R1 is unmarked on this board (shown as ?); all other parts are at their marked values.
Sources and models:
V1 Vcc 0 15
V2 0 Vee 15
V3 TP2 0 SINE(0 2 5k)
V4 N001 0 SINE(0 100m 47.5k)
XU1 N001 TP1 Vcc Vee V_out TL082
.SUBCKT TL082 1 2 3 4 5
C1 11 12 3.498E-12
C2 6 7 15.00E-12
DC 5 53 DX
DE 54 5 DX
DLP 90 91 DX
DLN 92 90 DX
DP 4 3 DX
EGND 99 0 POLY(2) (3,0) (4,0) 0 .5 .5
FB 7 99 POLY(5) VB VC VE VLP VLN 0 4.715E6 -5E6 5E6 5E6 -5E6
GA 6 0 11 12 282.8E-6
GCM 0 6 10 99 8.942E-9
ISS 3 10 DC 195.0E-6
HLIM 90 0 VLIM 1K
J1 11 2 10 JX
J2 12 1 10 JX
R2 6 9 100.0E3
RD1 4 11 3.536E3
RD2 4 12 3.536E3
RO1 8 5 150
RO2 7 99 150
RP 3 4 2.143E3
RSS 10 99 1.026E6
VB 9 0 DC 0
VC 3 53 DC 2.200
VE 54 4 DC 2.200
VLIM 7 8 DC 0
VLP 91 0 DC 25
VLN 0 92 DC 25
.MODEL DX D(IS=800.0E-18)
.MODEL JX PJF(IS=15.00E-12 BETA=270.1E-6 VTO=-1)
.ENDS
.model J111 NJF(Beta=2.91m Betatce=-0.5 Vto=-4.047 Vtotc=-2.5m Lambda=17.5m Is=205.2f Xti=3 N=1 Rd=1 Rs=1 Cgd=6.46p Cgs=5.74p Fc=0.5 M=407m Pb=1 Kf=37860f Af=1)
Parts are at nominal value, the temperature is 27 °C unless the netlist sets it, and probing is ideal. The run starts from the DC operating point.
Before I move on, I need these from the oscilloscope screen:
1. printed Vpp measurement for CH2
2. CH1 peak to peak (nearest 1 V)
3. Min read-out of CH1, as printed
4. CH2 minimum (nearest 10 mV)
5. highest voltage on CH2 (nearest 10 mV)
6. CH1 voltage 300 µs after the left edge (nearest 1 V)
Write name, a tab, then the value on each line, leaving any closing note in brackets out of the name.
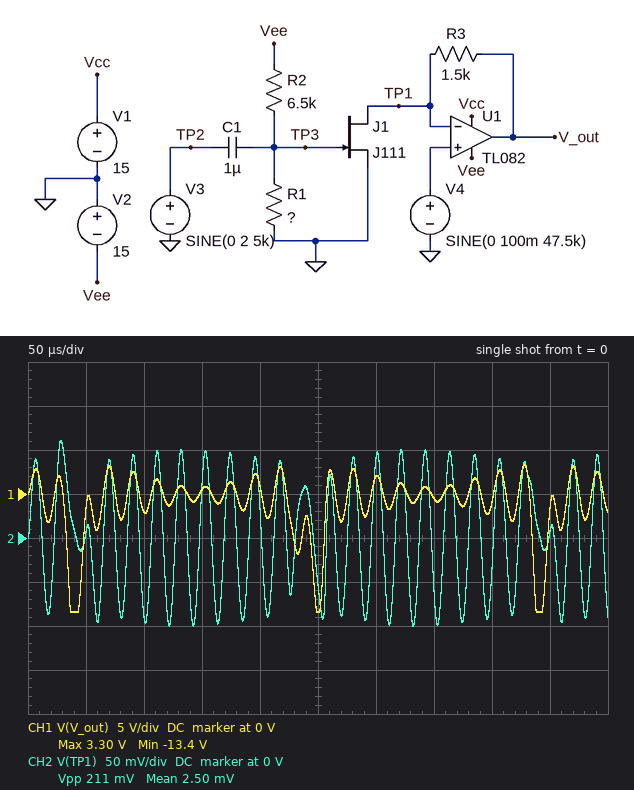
printed Vpp measurement for CH2	211 mV
CH1 peak to peak	17 V
Min read-out of CH1, as printed	-13.4 V
CH2 minimum	-100 mV
highest voltage on CH2	110 mV
CH1 voltage 300 µs after the left edge	2 V
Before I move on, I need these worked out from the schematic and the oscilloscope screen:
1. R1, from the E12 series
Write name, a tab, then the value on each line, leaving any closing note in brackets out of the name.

R1, from the E12 series	330 Ω
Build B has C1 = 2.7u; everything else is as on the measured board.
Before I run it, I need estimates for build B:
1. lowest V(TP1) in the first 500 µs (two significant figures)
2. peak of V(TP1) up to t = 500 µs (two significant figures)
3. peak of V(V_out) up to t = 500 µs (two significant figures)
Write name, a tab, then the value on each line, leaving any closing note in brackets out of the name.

lowest V(TP1) in the first 500 µs	-140 mV
peak of V(TP1) up to t = 500 µs	150 mV
peak of V(V_out) up to t = 500 µs	3.2 V
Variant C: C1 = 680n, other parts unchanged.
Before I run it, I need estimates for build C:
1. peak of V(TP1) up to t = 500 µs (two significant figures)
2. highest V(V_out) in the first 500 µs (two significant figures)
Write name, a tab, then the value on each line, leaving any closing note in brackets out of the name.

peak of V(TP1) up to t = 500 µs	100 mV
highest V(V_out) in the first 500 µs	3.2 V
